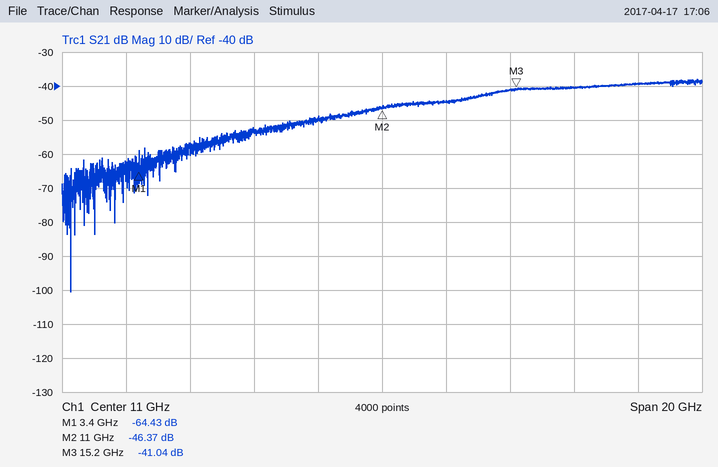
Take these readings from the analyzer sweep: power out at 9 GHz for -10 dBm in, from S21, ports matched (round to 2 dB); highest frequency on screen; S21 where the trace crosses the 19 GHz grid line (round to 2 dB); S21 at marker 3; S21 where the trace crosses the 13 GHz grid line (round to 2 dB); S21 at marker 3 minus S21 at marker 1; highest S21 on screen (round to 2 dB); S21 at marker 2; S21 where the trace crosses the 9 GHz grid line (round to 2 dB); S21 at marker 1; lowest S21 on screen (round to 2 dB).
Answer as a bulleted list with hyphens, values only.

- -60 dBm
- 21 GHz
- -40 dB
- -41.04 dB
- -44 dB
- 23.39 dB
- -38 dB
- -46.37 dB
- -50 dB
- -64.43 dB
- -100 dB
